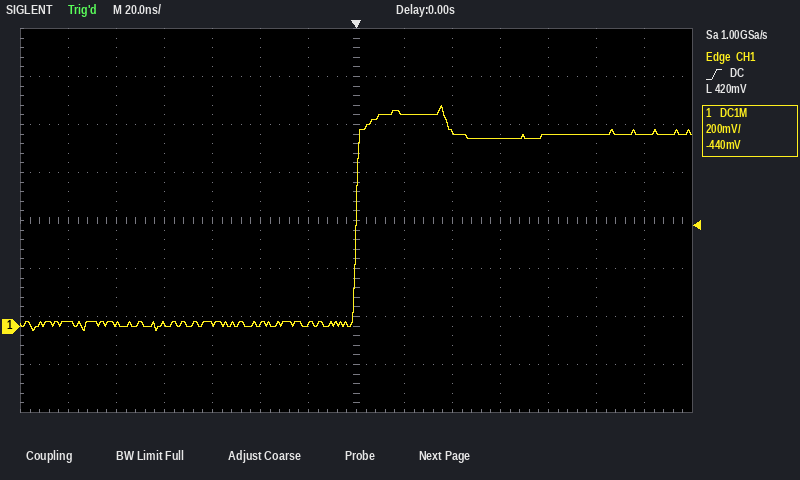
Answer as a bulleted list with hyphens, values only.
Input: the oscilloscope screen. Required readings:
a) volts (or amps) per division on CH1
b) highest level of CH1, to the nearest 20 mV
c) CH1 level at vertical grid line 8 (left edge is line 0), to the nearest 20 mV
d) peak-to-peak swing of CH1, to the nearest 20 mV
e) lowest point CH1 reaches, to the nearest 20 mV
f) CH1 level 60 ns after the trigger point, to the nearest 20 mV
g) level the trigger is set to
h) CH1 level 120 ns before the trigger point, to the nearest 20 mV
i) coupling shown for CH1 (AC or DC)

- 200 mV
- 920 mV
- 880 mV
- 940 mV
- -20 mV
- 780 mV
- 420 mV
- 20 mV
- DC
